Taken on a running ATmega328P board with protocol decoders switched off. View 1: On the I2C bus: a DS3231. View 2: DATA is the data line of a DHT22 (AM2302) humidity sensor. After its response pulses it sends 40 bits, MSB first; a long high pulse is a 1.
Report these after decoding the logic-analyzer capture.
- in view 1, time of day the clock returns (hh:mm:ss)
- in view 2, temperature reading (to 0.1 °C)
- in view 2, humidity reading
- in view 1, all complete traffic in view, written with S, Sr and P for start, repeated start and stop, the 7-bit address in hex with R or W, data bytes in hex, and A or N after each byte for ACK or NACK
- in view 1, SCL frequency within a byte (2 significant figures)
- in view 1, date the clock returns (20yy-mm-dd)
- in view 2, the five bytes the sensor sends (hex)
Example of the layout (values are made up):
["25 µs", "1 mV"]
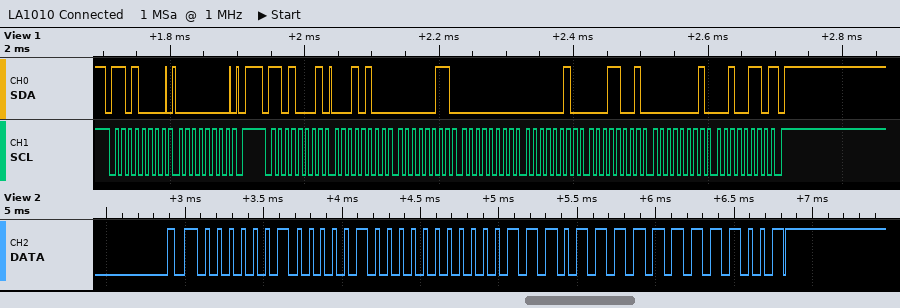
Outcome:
["00:03:14", "23.9 °C", "52.0 %", "S 68W A 00 A P S 68R A 14 A 03 A 00 A 02 A 19 A 01 A 26 N P", "100 kHz", "2026-01-19", "02 08 00 EF F9"]
